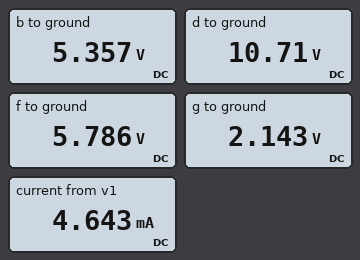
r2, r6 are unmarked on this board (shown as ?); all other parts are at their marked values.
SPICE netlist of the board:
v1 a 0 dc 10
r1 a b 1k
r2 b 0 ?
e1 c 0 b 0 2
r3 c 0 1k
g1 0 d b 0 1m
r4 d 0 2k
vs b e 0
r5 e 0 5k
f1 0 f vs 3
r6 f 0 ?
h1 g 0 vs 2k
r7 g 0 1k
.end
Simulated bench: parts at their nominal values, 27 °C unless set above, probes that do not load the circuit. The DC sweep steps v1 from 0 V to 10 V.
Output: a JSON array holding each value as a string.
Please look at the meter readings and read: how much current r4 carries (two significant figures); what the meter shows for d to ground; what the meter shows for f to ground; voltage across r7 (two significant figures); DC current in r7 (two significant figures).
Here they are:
["5.4 mA", "10.71 V", "5.786 V", "2.1 V", "2.1 mA"]
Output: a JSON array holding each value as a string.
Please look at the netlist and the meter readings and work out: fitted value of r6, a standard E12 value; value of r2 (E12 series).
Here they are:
["1.8 kΩ", "1.5 kΩ"]
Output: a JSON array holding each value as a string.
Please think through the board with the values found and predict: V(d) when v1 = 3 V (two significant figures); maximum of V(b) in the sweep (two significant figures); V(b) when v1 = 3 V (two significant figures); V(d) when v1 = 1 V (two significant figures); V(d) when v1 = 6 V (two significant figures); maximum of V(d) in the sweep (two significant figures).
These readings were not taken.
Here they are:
["3.2 V", "5.4 V", "1.6 V", "1.1 V", "6.4 V", "11 V"]
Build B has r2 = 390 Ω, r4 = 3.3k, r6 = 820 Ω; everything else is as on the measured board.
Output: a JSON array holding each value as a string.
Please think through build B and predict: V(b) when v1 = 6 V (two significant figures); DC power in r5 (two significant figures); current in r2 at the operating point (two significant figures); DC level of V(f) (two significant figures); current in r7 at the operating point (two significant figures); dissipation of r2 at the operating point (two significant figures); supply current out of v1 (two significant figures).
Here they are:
["1.6 V", "1.4 mW", "6.8 mA", "1.3 V", "1.1 mA", "18 mW", "7.3 mA"]
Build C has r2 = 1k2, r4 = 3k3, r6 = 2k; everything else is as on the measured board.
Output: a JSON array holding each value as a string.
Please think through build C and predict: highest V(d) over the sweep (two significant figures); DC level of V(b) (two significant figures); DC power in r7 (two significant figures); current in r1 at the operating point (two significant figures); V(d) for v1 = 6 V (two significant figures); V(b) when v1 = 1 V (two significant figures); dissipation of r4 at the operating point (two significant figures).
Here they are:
["16 V", "4.9 V", "3.9 mW", "5.1 mA", "9.7 V", "490 mV", "80 mW"]
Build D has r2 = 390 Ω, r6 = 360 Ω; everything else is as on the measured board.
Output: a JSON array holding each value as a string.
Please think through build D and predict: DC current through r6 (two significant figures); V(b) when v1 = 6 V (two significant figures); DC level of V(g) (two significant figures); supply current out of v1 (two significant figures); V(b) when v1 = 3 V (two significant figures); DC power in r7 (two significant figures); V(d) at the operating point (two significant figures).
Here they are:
["1.6 mA", "1.6 V", "1.1 V", "7.3 mA", "800 mV", "1.1 mW", "5.3 V"]
